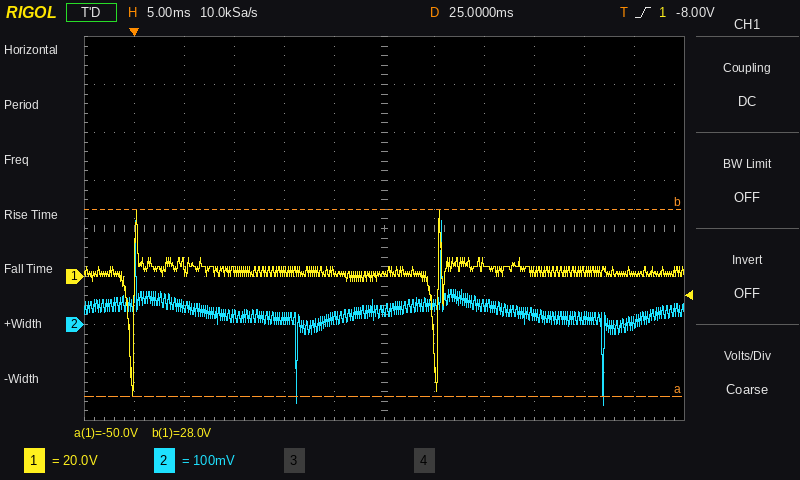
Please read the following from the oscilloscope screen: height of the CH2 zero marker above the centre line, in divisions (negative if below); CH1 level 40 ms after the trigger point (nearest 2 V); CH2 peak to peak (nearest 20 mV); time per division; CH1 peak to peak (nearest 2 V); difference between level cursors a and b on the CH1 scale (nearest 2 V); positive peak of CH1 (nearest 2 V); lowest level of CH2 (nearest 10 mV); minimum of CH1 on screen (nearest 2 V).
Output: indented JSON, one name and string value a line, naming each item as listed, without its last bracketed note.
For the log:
{
  "height of the CH2 zero marker above the centre line, in divisions": "-2.0 div",
  "CH1 level 40 ms after the trigger point": "2 V",
  "CH2 peak to peak": "380 mV",
  "time per division": "5 ms",
  "CH1 peak to peak": "78 V",
  "difference between level cursors a and b on the CH1 scale": "78 V",
  "positive peak of CH1": "28 V",
  "lowest level of CH2": "-170 mV",
  "minimum of CH1 on screen": "-50 V"
}
